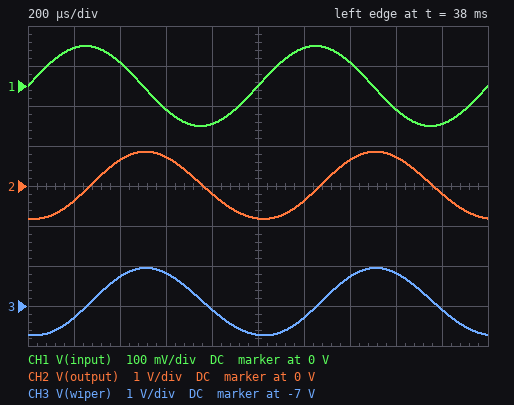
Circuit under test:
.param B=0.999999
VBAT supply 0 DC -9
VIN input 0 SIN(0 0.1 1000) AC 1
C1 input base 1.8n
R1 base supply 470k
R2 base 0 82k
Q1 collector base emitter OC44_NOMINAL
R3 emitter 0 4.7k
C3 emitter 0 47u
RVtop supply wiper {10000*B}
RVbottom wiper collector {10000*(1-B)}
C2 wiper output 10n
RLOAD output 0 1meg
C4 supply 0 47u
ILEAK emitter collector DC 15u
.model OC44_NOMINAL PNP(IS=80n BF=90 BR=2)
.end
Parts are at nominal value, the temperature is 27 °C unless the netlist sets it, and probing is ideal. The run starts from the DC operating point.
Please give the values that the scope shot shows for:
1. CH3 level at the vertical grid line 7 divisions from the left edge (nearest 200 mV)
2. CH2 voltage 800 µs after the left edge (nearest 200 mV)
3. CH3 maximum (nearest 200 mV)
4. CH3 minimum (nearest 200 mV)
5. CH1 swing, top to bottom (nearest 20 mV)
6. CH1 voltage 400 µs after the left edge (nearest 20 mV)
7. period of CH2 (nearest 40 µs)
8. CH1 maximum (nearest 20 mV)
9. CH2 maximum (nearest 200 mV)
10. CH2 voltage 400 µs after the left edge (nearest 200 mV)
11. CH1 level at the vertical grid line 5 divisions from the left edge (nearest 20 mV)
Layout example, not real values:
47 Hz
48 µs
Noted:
-6.2 V
-200 mV
-6.0 V
-7.8 V
200 mV
60 mV
1.00 ms
100 mV
800 mV
600 mV
0 V
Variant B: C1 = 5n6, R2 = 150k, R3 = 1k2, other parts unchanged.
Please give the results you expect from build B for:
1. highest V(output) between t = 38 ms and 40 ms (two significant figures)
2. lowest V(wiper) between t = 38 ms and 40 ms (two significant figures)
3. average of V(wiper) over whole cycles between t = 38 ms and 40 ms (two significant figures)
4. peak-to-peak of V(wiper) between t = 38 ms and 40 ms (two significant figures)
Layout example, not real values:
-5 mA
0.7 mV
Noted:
820 mV
-3.7 V
-1.8 V
2.6 V
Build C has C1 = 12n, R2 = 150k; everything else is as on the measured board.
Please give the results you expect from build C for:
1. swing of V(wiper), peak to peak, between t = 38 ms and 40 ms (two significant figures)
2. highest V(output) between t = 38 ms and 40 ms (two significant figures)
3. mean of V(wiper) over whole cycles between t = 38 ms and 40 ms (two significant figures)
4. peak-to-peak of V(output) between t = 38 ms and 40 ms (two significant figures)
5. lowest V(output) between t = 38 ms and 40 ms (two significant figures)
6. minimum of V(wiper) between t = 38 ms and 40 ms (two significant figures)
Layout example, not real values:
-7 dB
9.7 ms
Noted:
7.0 V
4.2 V
-5.8 V
7.1 V
-2.9 V
-8.7 V
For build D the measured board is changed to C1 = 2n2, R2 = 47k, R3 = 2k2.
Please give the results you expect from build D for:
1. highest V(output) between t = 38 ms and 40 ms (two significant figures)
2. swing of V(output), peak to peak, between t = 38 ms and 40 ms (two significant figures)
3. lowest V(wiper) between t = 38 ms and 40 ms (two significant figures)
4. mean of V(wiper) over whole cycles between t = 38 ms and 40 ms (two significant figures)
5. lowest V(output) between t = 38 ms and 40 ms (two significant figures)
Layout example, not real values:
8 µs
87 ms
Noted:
990 mV
1.9 V
-7.6 V
-6.7 V
-930 mV
